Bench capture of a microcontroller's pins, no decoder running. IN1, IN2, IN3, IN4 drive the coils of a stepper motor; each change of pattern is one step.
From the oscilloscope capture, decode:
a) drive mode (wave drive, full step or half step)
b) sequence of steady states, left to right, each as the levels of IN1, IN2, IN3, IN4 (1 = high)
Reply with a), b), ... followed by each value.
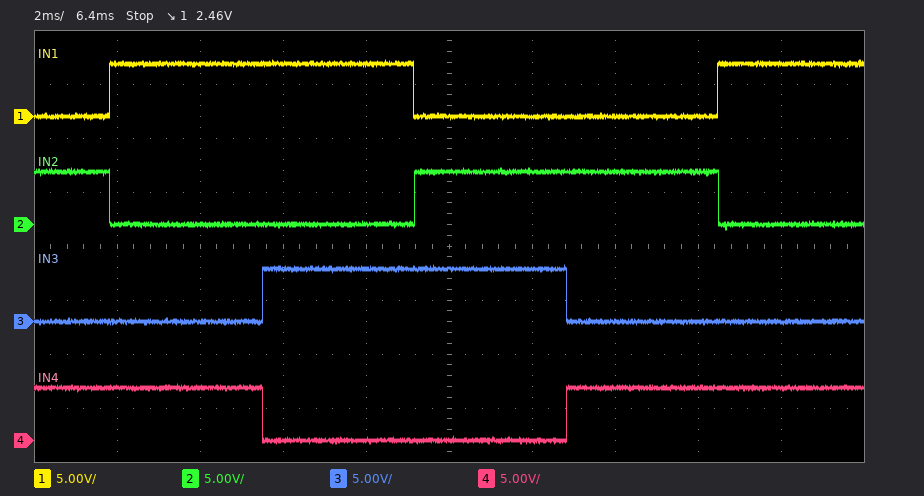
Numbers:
a) full step
b) 0101 1001 1010 0110 0101 1001
